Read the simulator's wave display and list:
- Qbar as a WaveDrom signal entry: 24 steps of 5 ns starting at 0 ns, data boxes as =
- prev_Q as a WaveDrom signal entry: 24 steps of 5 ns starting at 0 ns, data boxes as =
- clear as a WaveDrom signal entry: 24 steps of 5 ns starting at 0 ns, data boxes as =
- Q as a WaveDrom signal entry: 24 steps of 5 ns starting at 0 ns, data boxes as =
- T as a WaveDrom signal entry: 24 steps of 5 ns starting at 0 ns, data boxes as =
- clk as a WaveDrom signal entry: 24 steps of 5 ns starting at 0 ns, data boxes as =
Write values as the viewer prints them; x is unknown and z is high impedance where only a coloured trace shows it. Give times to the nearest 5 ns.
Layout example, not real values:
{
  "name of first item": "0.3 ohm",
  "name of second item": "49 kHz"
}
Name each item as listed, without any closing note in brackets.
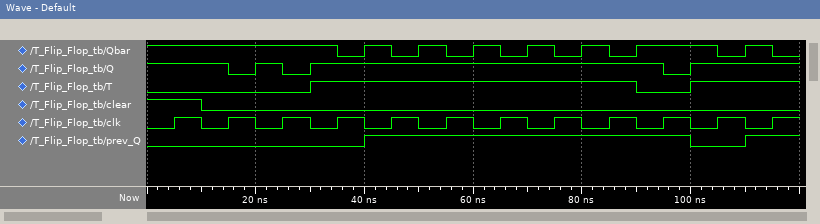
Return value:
{
  "Qbar as a WaveDrom signal entry: 24 steps of 5 ns starting at 0 ns, data boxes as =": "{name: 'Qbar', wave: '1......010101010101..010'}",
  "prev_Q as a WaveDrom signal entry: 24 steps of 5 ns starting at 0 ns, data boxes as =": "{name: 'prev_Q', wave: '0.......1...........0.1.'}",
  "clear as a WaveDrom signal entry: 24 steps of 5 ns starting at 0 ns, data boxes as =": "{name: 'clear', wave: '1.0.....................'}",
  "Q as a WaveDrom signal entry: 24 steps of 5 ns starting at 0 ns, data boxes as =": "{name: 'Q', wave: '1..0101............01...'}",
  "T as a WaveDrom signal entry: 24 steps of 5 ns starting at 0 ns, data boxes as =": "{name: 'T', wave: '0.....1...........0.1...'}",
  "clk as a WaveDrom signal entry: 24 steps of 5 ns starting at 0 ns, data boxes as =": "{name: 'clk', wave: '010101010101010101010101'}"
}
